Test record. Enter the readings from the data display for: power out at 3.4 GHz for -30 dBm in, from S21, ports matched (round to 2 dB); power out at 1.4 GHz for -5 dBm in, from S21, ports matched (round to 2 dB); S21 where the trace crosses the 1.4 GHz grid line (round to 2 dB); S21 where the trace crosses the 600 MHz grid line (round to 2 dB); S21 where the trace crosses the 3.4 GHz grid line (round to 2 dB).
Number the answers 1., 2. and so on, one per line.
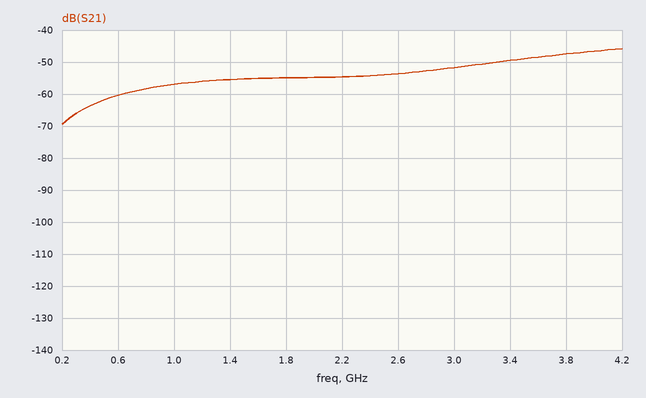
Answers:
1. -80 dBm
2. -60 dBm
3. -56 dB
4. -60 dB
5. -50 dB
